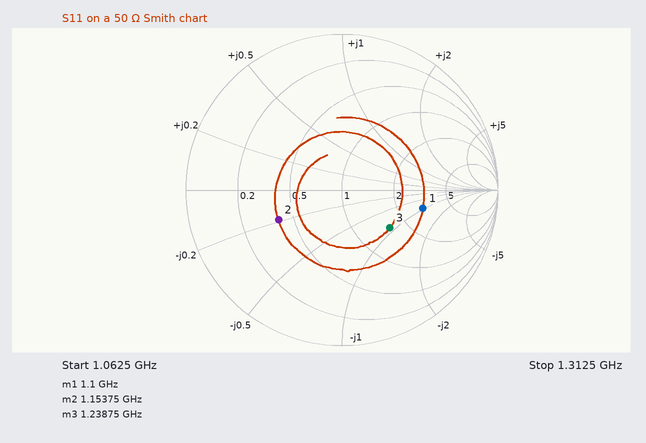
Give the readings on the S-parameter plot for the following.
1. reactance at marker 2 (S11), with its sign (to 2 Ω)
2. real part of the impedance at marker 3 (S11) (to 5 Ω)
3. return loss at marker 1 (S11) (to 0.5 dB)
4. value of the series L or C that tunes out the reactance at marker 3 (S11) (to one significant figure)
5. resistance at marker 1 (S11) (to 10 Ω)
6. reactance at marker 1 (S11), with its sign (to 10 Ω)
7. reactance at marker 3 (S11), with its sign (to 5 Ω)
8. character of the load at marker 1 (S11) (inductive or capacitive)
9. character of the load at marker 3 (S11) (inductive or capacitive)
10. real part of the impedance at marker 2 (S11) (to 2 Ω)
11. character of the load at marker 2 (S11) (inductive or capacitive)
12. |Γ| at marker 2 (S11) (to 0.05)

-10 Ω
80 Ω
5.5 dB
6 nH
150 Ω
-50 Ω
-45 Ω
capacitive
capacitive
20 Ω
capacitive
0.45
